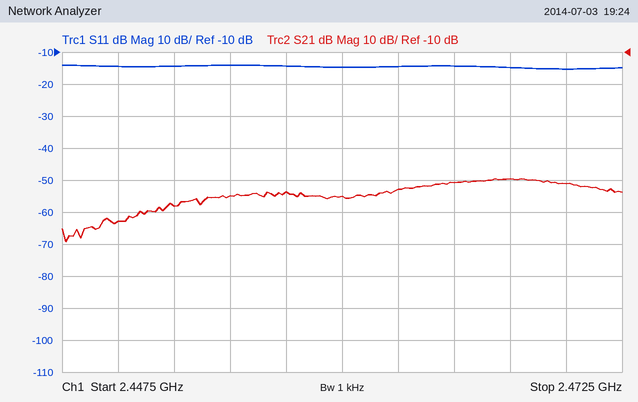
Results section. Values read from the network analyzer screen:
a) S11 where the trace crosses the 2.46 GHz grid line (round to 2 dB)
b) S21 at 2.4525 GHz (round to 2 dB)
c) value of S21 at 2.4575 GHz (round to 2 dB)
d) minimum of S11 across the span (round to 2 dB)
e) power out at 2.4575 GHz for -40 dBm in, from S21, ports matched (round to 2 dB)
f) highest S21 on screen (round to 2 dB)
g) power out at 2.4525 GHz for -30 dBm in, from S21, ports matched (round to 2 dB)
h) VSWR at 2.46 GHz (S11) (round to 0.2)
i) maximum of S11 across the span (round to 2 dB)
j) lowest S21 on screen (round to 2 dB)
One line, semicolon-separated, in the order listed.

-14 dB; -58 dB; -54 dB; -16 dB; -94 dBm; -50 dB; -88 dBm; 1.4; -14 dB; -70 dB
